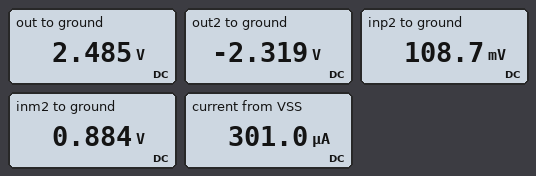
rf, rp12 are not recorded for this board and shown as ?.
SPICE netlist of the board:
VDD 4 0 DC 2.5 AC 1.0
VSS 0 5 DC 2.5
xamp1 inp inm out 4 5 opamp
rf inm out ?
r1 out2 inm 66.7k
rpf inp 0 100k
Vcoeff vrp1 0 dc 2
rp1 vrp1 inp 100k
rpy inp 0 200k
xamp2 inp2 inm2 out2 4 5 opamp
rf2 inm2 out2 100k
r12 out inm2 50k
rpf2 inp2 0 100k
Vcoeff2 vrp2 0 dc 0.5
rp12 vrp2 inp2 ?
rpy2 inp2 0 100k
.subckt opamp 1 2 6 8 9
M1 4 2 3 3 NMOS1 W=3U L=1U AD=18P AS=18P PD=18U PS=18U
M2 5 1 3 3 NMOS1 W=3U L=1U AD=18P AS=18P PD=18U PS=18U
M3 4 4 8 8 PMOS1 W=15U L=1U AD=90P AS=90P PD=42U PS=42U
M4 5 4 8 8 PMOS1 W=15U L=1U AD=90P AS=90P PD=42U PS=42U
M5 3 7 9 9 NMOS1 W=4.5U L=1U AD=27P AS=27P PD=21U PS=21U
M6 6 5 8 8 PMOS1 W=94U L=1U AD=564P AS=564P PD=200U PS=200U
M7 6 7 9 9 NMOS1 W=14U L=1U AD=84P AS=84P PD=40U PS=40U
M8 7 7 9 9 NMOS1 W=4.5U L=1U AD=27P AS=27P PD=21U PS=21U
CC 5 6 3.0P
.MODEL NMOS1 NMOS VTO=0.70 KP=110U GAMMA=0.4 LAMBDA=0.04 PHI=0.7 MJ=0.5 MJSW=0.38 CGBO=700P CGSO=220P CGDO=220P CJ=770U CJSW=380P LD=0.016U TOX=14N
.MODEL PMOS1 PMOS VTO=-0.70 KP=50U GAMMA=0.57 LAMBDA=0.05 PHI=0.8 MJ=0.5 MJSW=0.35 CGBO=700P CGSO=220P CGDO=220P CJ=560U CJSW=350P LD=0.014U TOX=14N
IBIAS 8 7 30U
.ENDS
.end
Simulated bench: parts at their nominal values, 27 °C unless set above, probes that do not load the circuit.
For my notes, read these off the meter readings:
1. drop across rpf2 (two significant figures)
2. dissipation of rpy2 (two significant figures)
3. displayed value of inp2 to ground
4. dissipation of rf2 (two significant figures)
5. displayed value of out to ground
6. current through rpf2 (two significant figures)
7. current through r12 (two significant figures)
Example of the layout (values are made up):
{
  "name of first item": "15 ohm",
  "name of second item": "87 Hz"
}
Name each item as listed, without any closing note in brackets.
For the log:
{
  "drop across rpf2": "110 mV",
  "dissipation of rpy2": "120 nW",
  "displayed value of inp2 to ground": "108.7 mV",
  "dissipation of rf2": "100 µW",
  "displayed value of out to ground": "2.485 V",
  "current through rpf2": "1.1 µA",
  "current through r12": "32 µA"
}
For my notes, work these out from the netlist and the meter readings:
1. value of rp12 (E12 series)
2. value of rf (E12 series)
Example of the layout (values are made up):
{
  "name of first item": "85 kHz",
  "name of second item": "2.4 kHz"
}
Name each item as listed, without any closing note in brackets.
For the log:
{
  "value of rp12": "180 kΩ",
  "value of rf": "56 kΩ"
}
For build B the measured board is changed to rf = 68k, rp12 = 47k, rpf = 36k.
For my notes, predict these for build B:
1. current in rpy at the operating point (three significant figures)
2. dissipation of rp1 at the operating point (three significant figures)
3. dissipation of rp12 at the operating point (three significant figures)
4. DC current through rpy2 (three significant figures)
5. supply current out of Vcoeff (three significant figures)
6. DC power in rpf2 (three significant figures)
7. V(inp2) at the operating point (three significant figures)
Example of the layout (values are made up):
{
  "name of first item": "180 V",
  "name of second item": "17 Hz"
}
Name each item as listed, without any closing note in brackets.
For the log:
{
  "current in rpy at the operating point": "2.34 µA",
  "dissipation of rp1 at the operating point": "23.5 µW",
  "dissipation of rp12 at the operating point": "1.25 µW",
  "DC current through rpy2": "2.58 µA",
  "supply current out of Vcoeff": "15.3 µA",
  "DC power in rpf2": "664 nW",
  "V(inp2) at the operating point": "258 mV"
}
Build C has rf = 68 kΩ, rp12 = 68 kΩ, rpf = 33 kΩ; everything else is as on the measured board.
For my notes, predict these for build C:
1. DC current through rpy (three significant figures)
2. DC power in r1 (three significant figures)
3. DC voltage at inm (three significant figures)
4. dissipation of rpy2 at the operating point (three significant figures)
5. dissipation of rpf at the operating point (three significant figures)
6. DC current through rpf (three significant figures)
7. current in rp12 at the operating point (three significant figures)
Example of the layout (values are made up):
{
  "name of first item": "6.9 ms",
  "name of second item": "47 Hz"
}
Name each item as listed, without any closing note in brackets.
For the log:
{
  "DC current through rpy": "2.21 µA",
  "DC power in r1": "85.3 µW",
  "DC voltage at inm": "54.2 mV",
  "dissipation of rpy2 at the operating point": "449 nW",
  "dissipation of rpf at the operating point": "5.91 µW",
  "DC current through rpf": "13.4 µA",
  "current in rp12 at the operating point": "4.24 µA"
}
